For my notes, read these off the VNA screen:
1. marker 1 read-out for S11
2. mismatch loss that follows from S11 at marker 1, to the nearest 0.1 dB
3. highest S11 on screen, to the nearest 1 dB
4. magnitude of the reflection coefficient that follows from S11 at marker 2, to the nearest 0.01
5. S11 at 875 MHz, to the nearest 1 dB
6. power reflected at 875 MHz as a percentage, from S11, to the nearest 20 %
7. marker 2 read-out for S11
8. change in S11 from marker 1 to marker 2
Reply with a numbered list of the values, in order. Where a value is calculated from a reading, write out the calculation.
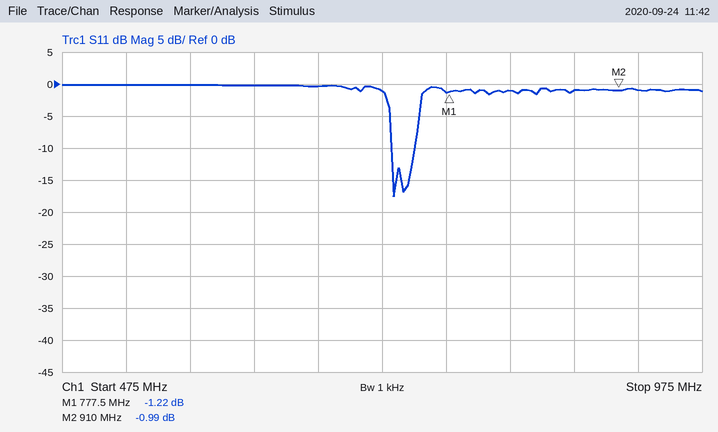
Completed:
1. -1.22 dB
2. −10 log10(1 − 10^(-1.22/10)) ≈ 6.1 dB
3. 0 dB
4. 10^(-0.99/20) ≈ 0.89
5. -1 dB
6. 10^(-1/10) ≈ 79.4 %, so 80 % to the nearest 20 %
7. -0.99 dB
8. -0.99 − (-1.22) = 0.23 dB
